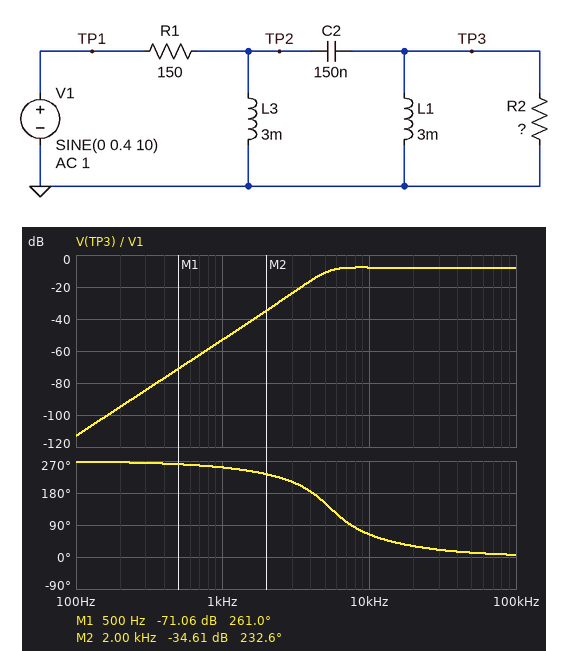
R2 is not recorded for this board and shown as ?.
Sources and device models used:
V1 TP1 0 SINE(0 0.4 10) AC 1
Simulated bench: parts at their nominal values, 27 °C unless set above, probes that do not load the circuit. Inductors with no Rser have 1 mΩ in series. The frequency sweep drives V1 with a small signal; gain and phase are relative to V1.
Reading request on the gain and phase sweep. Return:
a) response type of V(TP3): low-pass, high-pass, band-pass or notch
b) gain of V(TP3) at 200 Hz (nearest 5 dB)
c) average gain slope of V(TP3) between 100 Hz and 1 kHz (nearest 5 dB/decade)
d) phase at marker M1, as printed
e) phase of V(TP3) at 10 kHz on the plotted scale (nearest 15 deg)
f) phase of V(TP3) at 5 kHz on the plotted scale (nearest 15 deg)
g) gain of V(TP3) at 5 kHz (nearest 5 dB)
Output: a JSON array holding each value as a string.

["high-pass", "-95 dB", "60 dB/decade", "261.0 deg", "60 deg", "150 deg", "-10 dB"]
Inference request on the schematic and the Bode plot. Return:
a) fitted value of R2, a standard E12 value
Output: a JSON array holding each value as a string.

["100 Ω"]
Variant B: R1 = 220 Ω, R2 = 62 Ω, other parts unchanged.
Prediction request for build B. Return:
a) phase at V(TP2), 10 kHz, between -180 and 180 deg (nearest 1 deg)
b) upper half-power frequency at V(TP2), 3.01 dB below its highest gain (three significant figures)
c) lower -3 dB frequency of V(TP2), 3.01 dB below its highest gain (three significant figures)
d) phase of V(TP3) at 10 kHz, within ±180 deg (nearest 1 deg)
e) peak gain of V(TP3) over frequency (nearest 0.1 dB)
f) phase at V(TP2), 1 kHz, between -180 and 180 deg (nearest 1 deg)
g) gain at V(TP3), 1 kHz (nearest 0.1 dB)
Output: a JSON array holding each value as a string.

["-16 deg", "9.81 kHz", "4.17 kHz", "60 deg", "-11.6 dB", "85 deg", "-56.5 dB"]
